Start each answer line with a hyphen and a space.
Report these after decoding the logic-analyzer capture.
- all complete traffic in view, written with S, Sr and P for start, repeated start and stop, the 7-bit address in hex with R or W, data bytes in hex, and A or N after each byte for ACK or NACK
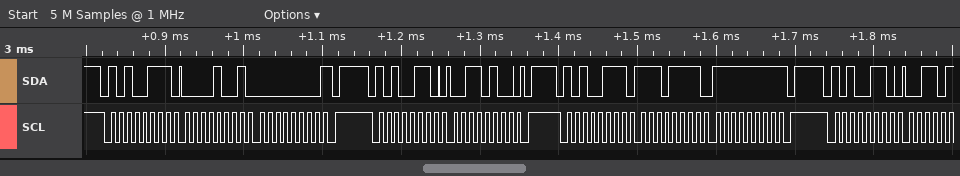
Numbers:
- S 53R A 09 A 00 N P S 53W A 34 A P S 53R A EF A FF N P S 53W A
